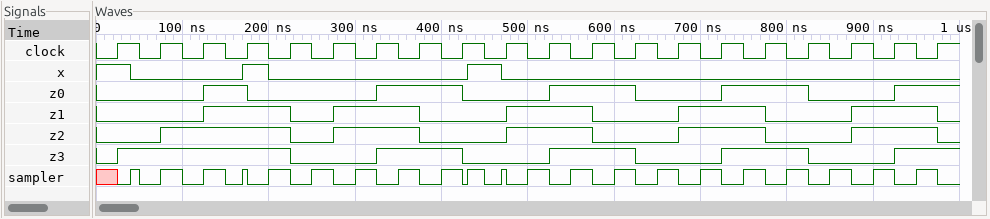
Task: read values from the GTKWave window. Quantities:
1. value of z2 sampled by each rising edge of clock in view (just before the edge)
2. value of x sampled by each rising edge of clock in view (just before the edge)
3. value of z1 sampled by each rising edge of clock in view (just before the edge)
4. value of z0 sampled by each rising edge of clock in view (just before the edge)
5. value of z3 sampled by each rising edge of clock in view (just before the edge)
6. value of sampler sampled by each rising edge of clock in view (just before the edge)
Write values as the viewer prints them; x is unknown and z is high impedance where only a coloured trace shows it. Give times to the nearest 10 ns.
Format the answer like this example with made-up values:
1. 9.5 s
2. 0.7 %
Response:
1. 0 0 1 1 1 0 1 1 0 0 1 1 0 0 1 1 0 0 1 1
2. 1 0 0 1 0 0 0 0 0 0 0 0 0 0 0 0 0 0 0 0
3. 0 0 0 1 1 0 1 1 0 0 1 1 0 0 1 1 0 0 1 1
4. 0 0 0 1 0 0 0 1 1 0 0 1 1 0 0 1 1 0 0 1
5. 0 1 1 1 1 0 0 1 1 0 0 1 1 0 0 1 1 0 0 1
6. x 0 0 1 1 1 1 1 1 1 1 1 1 1 1 1 1 1 1 1
